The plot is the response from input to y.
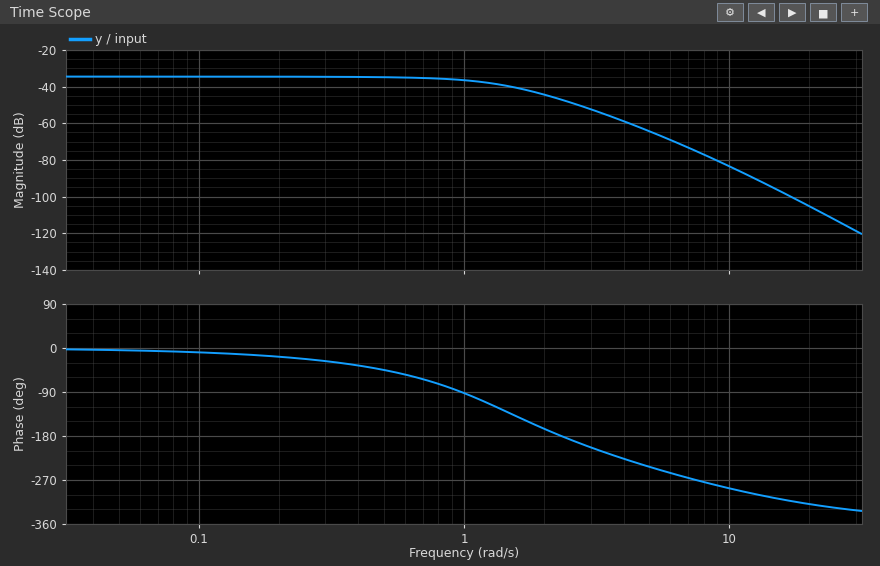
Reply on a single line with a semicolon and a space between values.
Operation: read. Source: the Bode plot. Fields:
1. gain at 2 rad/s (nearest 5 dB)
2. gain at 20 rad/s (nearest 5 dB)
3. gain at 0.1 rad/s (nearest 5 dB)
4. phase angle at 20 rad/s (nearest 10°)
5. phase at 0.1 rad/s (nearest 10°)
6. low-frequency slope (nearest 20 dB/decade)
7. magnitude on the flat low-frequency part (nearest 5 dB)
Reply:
-45 dB; -105 dB; -35 dB; -320°; -10°; 0 dB/decade; -35 dB
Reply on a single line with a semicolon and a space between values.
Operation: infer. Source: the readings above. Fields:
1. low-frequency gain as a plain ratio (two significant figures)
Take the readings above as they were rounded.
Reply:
0.018
